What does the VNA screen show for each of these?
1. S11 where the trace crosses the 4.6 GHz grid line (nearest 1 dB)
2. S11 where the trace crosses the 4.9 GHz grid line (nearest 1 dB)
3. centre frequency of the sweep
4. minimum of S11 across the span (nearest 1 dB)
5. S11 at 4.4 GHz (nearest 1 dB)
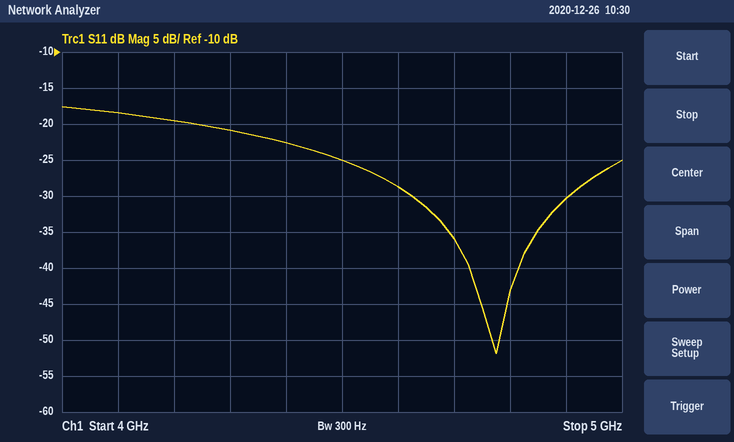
-29 dB
-30 dB
4.5 GHz
-52 dB
-23 dB
